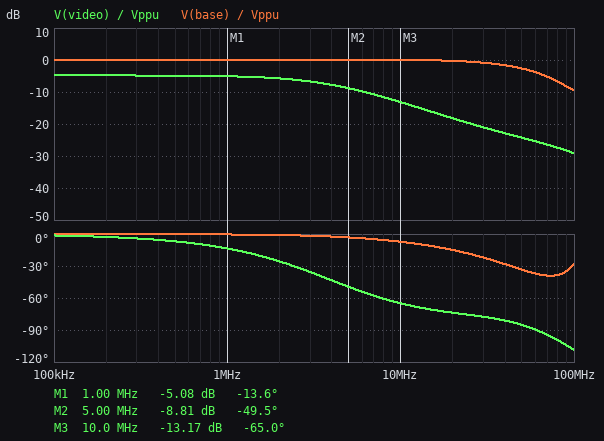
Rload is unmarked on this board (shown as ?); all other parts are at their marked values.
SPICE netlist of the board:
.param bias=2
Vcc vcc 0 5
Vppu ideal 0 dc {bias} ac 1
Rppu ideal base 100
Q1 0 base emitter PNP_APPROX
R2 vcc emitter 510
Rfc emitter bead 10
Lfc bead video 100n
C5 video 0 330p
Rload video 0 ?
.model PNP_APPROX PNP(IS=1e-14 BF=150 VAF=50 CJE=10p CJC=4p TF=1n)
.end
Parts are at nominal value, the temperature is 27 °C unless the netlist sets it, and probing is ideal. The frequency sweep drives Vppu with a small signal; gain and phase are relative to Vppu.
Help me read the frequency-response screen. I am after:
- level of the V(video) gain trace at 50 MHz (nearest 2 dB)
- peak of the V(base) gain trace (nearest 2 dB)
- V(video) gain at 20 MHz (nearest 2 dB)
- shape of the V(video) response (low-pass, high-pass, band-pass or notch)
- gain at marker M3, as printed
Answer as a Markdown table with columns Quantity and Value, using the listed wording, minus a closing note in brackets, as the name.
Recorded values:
| Quantity | Value |
|---|---|
| level of the V(video) gain trace at 50 MHz | -24 dB |
| peak of the V(base) gain trace | 0 dB |
| V(video) gain at 20 MHz | -18 dB |
| shape of the V(video) response | low-pass |
| gain at marker M3, as printed | -13.17 dB |
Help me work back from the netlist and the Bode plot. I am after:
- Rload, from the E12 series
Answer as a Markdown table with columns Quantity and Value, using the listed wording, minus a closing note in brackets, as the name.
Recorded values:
| Quantity | Value |
|---|---|
| Rload, from the E12 series | 560 Ω |
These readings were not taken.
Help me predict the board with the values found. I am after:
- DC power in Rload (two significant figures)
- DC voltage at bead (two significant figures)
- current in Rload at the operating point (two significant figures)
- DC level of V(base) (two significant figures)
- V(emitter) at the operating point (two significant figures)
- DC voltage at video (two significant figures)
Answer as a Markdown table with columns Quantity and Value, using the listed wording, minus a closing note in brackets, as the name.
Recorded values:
| Quantity | Value |
|---|---|
| DC power in Rload | 12 mW |
| DC voltage at bead | 2.6 V |
| current in Rload at the operating point | 4.6 mA |
| DC level of V(base) | 2.0 V |
| V(emitter) at the operating point | 2.6 V |
| DC voltage at video | 2.6 V |
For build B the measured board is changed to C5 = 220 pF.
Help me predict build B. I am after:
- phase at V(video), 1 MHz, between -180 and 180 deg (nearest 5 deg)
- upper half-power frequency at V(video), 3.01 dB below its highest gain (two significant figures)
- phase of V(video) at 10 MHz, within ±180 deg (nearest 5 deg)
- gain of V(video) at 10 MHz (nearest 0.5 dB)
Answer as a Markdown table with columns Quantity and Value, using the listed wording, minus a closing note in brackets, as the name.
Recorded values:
| Quantity | Value |
|---|---|
| phase at V(video), 1 MHz, between -180 and 180 deg | -10 deg |
| upper half-power frequency at V(video), 3.01 dB below its highest gain | 6.1 MHz |
| phase of V(video) at 10 MHz, within ±180 deg | -55 deg |
| gain of V(video) at 10 MHz | -10.5 dB |
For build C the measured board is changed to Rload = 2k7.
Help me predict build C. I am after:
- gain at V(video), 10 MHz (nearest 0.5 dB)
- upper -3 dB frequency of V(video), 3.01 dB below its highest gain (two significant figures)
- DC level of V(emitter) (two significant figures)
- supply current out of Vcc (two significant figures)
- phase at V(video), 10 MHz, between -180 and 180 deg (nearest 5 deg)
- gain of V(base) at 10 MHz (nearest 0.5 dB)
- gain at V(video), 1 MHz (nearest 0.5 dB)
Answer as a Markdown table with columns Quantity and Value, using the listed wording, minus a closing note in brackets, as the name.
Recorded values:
| Quantity | Value |
|---|---|
| gain at V(video), 10 MHz | 1.5 dB |
| upper -3 dB frequency of V(video), 3.01 dB below its highest gain | 23 MHz |
| DC level of V(emitter) | 2.7 V |
| supply current out of Vcc | 4.5 mA |
| phase at V(video), 10 MHz, between -180 and 180 deg | -30 deg |
| gain of V(base) at 10 MHz | 1.0 dB |
| gain at V(video), 1 MHz | 0 dB |
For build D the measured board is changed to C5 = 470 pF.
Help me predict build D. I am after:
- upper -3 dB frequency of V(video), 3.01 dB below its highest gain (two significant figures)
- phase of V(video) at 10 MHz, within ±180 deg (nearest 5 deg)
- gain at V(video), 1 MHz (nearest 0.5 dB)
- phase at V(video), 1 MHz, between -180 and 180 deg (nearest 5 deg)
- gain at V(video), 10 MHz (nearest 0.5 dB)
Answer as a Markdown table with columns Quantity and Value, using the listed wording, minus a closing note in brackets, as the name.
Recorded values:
| Quantity | Value |
|---|---|
| upper -3 dB frequency of V(video), 3.01 dB below its highest gain | 2.9 MHz |
| phase of V(video) at 10 MHz, within ±180 deg | -70 deg |
| gain at V(video), 1 MHz | -5.5 dB |
| phase at V(video), 1 MHz, between -180 and 180 deg | -20 deg |
| gain at V(video), 10 MHz | -16.0 dB |
